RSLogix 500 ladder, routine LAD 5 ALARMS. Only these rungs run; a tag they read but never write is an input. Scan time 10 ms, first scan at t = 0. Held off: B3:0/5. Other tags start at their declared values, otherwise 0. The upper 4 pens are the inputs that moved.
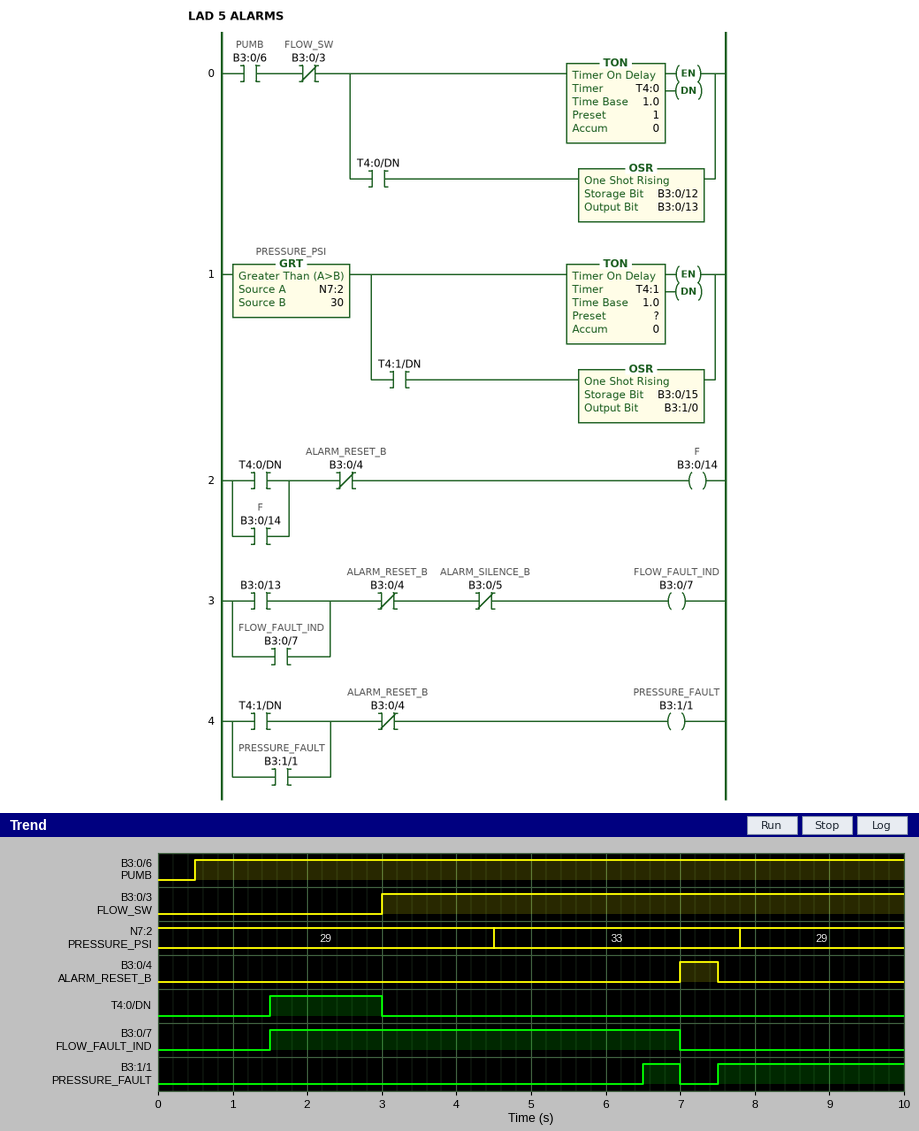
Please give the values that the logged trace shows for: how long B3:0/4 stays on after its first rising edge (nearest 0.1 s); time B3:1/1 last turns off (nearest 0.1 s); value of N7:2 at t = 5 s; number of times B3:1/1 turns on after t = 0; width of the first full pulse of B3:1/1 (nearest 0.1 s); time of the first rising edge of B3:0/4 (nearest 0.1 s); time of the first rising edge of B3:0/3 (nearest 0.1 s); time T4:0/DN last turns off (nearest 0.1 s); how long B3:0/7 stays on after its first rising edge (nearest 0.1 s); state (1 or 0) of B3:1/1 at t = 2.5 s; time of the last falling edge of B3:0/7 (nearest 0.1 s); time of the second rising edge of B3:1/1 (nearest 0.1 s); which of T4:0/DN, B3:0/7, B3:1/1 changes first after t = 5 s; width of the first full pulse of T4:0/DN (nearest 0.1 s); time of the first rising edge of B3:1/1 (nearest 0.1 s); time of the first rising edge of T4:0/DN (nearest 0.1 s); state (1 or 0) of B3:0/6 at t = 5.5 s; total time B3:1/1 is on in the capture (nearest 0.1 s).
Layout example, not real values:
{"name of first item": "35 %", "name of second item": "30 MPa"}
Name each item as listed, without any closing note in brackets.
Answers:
{"how long B3:0/4 stays on after its first rising edge": "0.5 s", "time B3:1/1 last turns off": "7.0 s", "value of N7:2 at t = 5 s": "33", "number of times B3:1/1 turns on after t = 0": "2", "width of the first full pulse of B3:1/1": "0.5 s", "time of the first rising edge of B3:0/4": "7.0 s", "time of the first rising edge of B3:0/3": "3.0 s", "time T4:0/DN last turns off": "3.0 s", "how long B3:0/7 stays on after its first rising edge": "5.5 s", "state (1 or 0) of B3:1/1 at t = 2.5 s": "0", "time of the last falling edge of B3:0/7": "7.0 s", "time of the second rising edge of B3:1/1": "7.5 s", "which of T4:0/DN, B3:0/7, B3:1/1 changes first after t = 5 s": "B3:1/1", "width of the first full pulse of T4:0/DN": "1.5 s", "time of the first rising edge of B3:1/1": "6.5 s", "time of the first rising edge of T4:0/DN": "1.5 s", "state (1 or 0) of B3:0/6 at t = 5.5 s": "1", "total time B3:1/1 is on in the capture": "3.0 s"}
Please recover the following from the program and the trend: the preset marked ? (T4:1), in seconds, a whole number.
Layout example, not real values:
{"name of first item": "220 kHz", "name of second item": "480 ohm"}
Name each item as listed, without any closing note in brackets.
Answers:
{"the preset marked ? (T4:1), in seconds, a whole number": "2 s"}
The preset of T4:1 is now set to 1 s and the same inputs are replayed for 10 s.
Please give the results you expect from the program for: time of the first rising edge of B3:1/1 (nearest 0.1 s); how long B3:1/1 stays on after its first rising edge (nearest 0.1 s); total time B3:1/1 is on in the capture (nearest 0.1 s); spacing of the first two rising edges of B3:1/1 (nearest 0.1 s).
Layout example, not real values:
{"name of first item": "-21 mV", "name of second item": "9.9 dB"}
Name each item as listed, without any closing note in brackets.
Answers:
{"time of the first rising edge of B3:1/1": "5.5 s", "how long B3:1/1 stays on after its first rising edge": "1.5 s", "total time B3:1/1 is on in the capture": "4.0 s", "spacing of the first two rising edges of B3:1/1": "2.0 s"}
